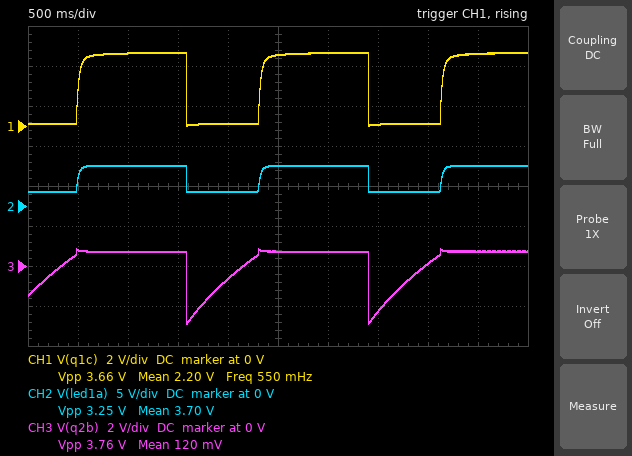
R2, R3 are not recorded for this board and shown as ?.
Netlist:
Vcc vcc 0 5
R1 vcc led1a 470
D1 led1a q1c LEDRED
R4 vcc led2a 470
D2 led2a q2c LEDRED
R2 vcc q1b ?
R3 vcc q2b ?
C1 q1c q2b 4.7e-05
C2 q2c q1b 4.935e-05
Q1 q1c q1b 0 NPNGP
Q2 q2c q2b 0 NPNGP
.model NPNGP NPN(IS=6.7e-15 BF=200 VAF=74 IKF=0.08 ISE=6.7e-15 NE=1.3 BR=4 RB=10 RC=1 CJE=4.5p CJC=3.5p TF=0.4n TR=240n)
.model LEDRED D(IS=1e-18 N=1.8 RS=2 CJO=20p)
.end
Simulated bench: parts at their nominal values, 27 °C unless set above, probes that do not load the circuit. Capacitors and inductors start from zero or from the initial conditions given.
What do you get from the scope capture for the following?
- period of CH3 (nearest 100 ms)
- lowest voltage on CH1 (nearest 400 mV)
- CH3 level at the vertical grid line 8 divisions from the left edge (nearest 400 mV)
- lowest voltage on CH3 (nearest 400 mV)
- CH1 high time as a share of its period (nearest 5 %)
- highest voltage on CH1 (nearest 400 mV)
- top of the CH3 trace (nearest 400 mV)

1.8 s
0 V
0 V
-2.8 V
60 %
3.6 V
800 mV
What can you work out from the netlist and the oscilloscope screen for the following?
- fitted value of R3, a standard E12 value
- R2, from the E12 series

27 kΩ
39 kΩ
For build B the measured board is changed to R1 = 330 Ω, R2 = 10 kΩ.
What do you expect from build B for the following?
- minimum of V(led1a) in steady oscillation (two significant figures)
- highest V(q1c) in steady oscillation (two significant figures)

1.8 V
3.6 V
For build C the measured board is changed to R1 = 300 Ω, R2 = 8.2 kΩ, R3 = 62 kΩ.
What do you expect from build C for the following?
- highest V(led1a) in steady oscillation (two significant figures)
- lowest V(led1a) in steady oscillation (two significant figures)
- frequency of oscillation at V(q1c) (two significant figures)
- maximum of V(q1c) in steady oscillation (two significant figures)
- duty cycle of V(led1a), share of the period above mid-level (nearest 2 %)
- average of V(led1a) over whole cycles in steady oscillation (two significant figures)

5.0 V
1.8 V
530 mHz
3.6 V
12 %
2.2 V
